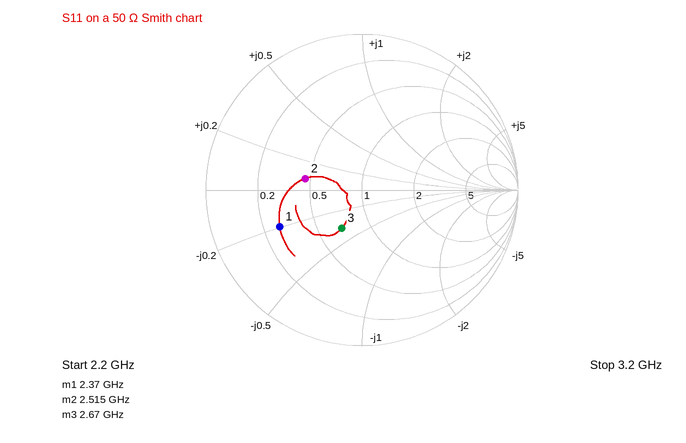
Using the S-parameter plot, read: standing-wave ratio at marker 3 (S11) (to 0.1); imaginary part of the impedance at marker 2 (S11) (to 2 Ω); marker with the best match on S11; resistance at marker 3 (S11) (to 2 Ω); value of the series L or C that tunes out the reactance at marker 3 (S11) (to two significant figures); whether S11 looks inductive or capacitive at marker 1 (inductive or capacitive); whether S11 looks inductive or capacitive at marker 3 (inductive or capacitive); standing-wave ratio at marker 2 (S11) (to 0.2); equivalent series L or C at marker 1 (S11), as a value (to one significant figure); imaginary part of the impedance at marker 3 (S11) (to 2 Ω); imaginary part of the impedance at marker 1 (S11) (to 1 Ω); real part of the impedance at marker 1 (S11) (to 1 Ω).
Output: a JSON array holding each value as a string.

["1.8", "+4 Ω", "marker 3", "34 Ω", "1.1 nH", "capacitive", "capacitive", "2.2", "7 pF", "-18 Ω", "-10 Ω", "14 Ω"]
